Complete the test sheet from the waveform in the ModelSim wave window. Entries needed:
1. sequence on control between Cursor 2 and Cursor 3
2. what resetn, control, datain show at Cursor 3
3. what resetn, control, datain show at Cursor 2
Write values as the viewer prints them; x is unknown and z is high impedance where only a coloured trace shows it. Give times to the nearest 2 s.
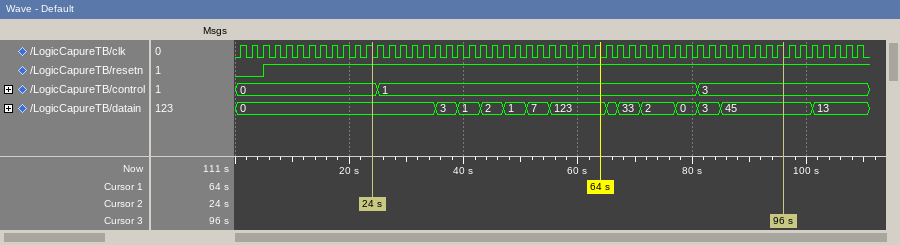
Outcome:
0, 1, 3
resetn=1, control=3, datain=45
resetn=1, control=0, datain=0
